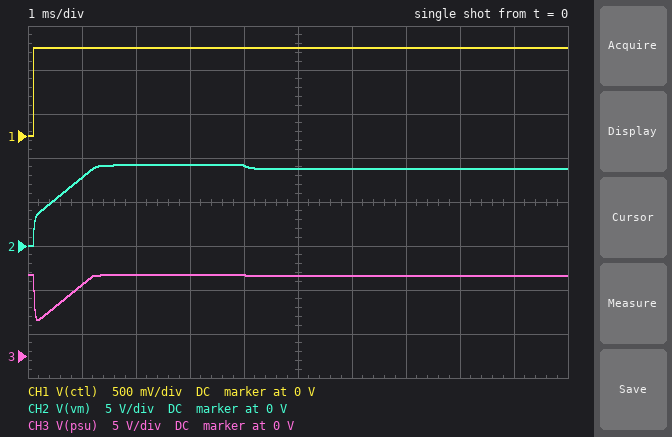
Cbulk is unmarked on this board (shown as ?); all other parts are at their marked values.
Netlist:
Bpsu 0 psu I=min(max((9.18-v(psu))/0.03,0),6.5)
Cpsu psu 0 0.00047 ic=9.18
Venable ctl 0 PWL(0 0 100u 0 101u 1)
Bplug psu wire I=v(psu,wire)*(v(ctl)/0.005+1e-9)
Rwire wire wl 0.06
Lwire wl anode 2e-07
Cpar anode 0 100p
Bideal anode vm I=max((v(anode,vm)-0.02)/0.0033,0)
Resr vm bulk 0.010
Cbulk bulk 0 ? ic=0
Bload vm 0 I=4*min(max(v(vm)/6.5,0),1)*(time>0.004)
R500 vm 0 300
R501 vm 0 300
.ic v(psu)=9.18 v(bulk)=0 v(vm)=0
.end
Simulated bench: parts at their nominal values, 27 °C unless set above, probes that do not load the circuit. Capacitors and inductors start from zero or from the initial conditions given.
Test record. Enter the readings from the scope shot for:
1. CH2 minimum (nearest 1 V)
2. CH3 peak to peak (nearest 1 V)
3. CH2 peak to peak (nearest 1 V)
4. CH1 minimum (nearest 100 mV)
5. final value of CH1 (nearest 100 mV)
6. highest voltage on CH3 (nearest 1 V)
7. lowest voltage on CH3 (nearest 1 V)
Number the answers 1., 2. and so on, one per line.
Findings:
1. 0 V
2. 5 V
3. 9 V
4. 0 V
5. 1.0 V
6. 9 V
7. 4 V
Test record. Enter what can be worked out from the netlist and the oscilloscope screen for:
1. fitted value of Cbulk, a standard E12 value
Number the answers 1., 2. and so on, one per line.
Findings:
1. 820 µF
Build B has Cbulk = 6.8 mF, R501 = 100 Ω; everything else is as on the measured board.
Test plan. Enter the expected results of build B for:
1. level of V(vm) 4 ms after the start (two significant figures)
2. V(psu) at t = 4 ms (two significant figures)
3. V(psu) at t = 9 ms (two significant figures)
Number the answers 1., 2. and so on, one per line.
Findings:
1. 4.1 V
2. 4.5 V
3. 6.7 V
